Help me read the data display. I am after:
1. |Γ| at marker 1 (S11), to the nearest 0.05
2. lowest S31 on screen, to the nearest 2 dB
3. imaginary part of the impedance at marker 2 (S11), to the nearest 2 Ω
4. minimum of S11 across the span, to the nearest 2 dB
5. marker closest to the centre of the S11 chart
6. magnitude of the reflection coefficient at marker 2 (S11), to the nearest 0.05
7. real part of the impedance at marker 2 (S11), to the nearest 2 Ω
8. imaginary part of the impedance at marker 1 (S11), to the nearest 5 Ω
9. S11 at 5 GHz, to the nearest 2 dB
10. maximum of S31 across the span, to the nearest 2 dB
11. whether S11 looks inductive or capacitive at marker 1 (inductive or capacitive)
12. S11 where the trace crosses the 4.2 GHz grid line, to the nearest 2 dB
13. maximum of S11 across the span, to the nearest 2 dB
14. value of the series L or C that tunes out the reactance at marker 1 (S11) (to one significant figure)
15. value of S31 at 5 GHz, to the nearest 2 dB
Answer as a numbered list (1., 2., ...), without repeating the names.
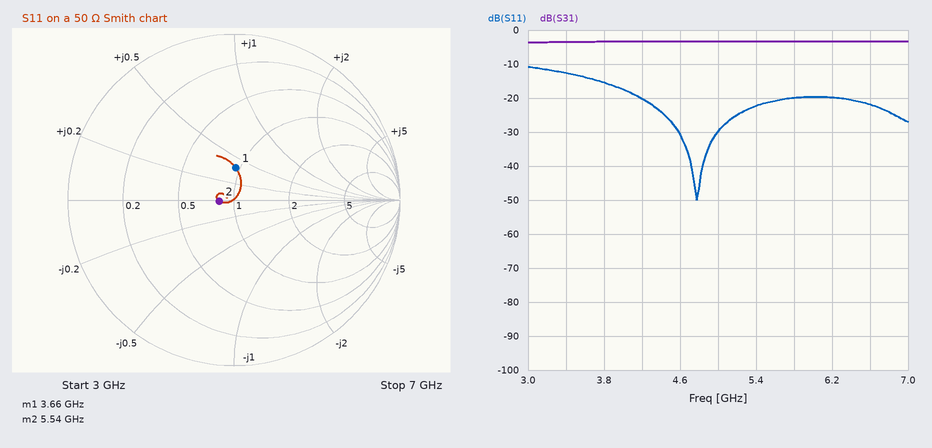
1. 0.20
2. -4 dB
3. 0 Ω
4. -50 dB
5. marker 2
6. 0.10
7. 42 Ω
8. +20 Ω
9. -30 dB
10. -4 dB
11. inductive
12. -20 dB
13. -10 dB
14. 2 pF
15. -4 dB
